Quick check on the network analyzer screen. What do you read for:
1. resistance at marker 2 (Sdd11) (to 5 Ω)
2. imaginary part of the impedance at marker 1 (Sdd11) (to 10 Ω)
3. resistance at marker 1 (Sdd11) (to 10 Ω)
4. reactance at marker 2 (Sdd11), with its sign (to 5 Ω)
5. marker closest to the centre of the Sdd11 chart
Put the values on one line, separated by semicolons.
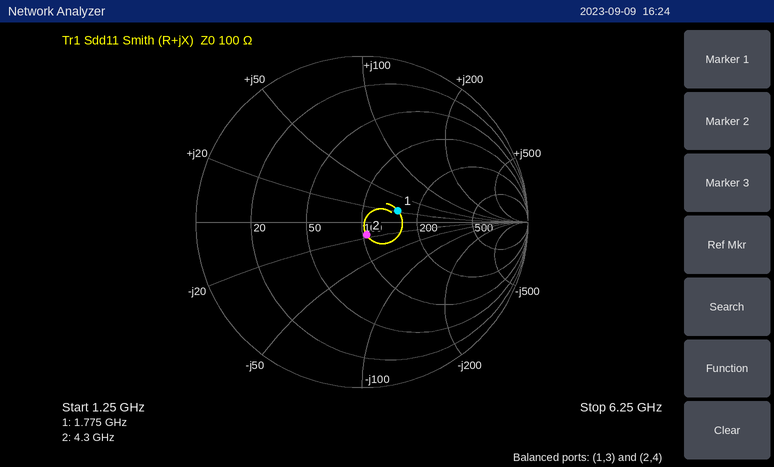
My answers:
105 Ω; +20 Ω; 150 Ω; -15 Ω; marker 2
